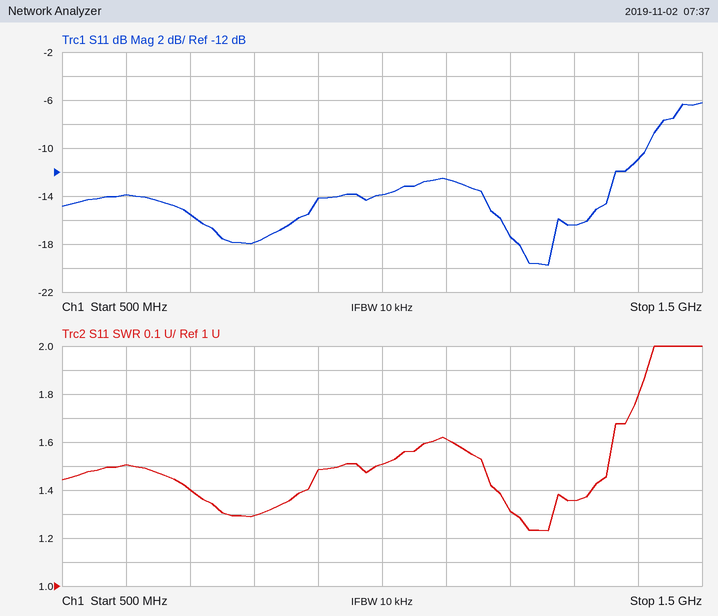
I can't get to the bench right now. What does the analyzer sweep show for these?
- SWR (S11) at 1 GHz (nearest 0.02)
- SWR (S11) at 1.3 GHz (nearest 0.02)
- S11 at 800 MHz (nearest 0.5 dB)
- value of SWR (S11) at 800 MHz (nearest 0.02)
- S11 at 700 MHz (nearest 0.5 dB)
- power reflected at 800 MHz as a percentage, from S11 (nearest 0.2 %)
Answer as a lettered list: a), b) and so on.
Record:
a) 1.50
b) 1.36
c) -18.0 dB
d) 1.30
e) -15.5 dB
f) 1.6 %
